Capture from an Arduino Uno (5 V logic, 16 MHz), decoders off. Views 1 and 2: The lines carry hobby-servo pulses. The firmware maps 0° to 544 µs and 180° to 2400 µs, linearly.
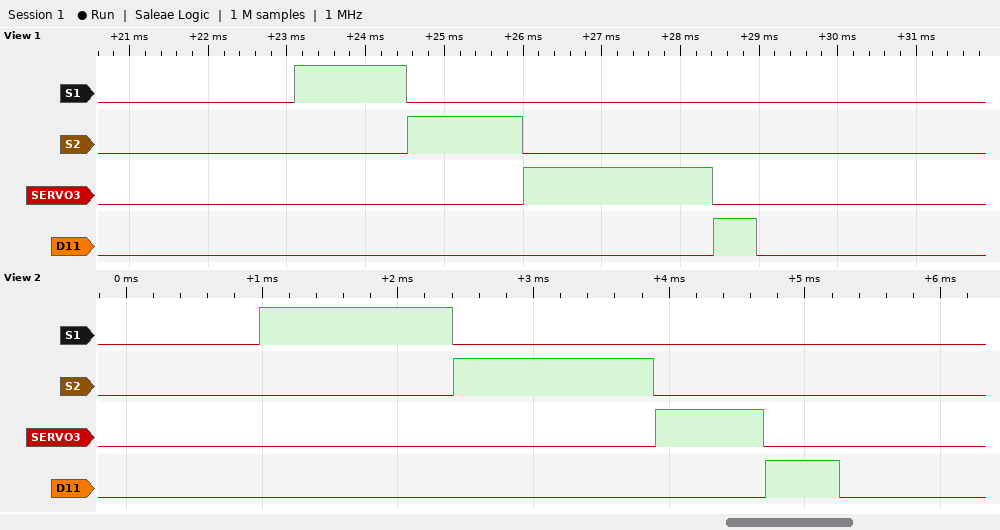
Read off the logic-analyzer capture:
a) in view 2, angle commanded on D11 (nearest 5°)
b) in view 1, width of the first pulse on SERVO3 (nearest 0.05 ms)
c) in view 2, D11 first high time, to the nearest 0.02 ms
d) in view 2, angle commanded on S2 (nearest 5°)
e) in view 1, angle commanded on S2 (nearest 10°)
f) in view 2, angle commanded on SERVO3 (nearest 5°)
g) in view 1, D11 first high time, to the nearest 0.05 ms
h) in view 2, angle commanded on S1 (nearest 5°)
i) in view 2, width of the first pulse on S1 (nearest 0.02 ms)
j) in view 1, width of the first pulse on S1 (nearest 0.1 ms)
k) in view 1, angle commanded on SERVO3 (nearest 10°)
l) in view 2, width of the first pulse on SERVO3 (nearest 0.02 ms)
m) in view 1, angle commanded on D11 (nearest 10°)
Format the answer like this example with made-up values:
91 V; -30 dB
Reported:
0°; 2.40 ms; 0.54 ms; 90°; 90°; 25°; 0.55 ms; 85°; 1.42 ms; 1.4 ms; 180°; 0.80 ms; 0°
